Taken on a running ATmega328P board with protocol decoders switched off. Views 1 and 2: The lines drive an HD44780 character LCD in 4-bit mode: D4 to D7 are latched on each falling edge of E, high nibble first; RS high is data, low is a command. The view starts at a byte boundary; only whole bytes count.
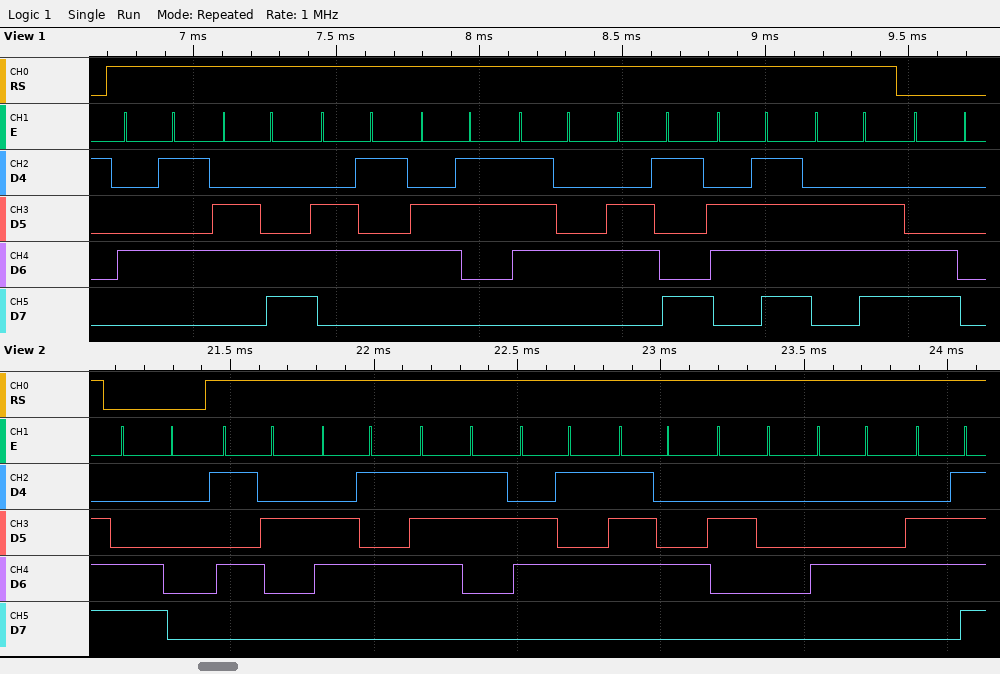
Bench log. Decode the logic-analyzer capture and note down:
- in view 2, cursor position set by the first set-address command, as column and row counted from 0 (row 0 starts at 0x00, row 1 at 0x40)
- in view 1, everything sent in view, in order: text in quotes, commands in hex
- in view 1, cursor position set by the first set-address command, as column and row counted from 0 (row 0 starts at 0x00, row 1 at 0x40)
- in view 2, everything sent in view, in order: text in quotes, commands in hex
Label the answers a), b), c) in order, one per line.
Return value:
a) column 0, row 1
b) "Election" 0xC0
c) column 0, row 1
d) 0xC0 "Reset Do"
